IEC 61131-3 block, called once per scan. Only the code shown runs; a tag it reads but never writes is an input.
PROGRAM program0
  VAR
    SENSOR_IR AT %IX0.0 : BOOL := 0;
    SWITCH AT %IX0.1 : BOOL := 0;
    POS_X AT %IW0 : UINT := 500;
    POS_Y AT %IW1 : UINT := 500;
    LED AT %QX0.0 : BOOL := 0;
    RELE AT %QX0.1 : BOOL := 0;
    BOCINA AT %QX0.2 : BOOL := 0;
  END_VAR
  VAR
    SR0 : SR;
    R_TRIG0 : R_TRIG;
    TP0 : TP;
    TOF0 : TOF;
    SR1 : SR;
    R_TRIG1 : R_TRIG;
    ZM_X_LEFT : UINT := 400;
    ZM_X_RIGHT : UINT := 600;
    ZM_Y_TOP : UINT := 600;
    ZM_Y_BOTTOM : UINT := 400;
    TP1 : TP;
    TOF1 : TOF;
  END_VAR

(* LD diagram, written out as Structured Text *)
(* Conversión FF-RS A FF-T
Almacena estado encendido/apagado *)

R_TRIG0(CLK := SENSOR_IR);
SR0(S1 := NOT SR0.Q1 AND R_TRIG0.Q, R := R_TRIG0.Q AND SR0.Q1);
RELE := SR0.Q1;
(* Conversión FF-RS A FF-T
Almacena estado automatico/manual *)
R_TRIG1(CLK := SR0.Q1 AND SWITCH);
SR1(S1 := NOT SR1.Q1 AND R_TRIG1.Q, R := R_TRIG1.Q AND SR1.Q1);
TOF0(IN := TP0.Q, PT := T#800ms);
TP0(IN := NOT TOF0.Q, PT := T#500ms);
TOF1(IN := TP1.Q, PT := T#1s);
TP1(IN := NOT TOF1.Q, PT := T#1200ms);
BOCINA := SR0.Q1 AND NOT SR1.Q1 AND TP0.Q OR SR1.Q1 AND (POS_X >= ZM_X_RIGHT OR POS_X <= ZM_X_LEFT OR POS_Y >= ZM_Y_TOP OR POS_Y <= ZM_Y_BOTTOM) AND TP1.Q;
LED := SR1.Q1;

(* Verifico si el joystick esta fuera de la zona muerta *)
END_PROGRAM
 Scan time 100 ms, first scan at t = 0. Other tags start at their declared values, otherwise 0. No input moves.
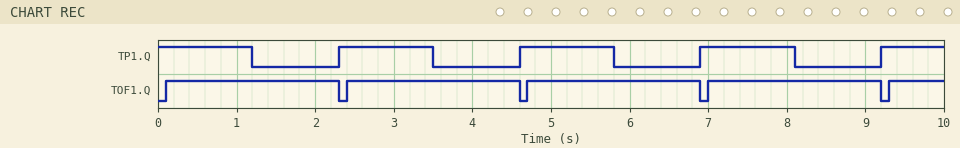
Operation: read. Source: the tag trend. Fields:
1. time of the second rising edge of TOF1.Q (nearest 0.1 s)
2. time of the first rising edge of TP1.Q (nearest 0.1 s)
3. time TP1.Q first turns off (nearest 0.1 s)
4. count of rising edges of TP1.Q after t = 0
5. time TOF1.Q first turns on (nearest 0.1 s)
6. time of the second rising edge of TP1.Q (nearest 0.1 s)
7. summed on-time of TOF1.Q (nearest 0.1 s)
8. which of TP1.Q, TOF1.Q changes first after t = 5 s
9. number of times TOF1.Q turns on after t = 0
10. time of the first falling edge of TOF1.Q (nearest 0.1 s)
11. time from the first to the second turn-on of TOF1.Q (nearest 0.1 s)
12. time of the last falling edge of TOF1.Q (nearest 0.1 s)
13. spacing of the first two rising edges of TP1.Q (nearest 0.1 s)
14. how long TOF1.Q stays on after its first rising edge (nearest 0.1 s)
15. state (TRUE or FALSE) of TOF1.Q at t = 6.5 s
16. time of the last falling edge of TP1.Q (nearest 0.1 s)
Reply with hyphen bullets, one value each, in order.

- 2.4 s
- 2.3 s
- 1.2 s
- 4
- 0.1 s
- 4.6 s
- 9.5 s
- TP1.Q
- 5
- 2.3 s
- 2.3 s
- 9.2 s
- 2.3 s
- 2.2 s
- TRUE
- 8.1 s
